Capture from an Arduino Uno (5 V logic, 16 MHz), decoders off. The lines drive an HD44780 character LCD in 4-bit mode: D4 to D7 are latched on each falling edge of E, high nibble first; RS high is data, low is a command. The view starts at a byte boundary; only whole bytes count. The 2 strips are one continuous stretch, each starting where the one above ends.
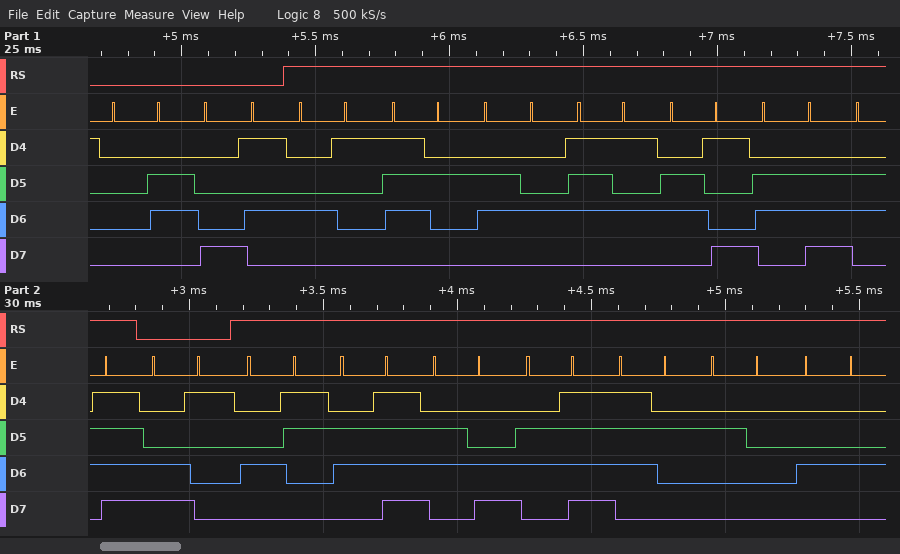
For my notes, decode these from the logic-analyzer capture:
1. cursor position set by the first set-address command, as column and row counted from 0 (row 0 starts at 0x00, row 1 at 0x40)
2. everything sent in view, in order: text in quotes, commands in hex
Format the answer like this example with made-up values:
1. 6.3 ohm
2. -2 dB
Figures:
1. column 5, row 0
2. 0x06 0x85 "Arduino" 0xC1 "Color D"
